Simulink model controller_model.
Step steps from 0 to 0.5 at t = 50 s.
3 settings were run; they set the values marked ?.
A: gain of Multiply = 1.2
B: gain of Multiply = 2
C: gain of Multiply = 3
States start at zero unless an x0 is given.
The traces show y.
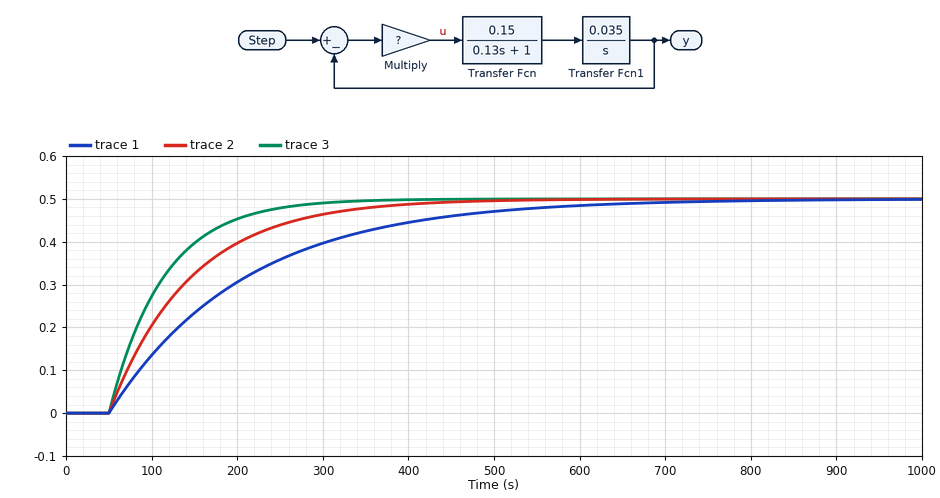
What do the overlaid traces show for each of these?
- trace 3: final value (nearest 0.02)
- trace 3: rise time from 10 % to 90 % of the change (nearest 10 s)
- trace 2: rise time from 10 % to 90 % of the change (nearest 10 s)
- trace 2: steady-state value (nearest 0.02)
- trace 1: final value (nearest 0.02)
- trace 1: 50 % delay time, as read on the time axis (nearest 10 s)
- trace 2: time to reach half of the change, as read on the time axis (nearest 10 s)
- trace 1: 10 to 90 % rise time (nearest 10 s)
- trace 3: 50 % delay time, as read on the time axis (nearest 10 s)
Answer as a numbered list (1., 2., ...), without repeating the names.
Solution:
1. 0.50
2. 140 s
3. 210 s
4. 0.50
5. 0.50
6. 160 s
7. 120 s
8. 350 s
9. 90 s
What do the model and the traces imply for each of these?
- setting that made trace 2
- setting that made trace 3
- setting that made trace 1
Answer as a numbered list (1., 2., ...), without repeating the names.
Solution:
1. B
2. C
3. A
